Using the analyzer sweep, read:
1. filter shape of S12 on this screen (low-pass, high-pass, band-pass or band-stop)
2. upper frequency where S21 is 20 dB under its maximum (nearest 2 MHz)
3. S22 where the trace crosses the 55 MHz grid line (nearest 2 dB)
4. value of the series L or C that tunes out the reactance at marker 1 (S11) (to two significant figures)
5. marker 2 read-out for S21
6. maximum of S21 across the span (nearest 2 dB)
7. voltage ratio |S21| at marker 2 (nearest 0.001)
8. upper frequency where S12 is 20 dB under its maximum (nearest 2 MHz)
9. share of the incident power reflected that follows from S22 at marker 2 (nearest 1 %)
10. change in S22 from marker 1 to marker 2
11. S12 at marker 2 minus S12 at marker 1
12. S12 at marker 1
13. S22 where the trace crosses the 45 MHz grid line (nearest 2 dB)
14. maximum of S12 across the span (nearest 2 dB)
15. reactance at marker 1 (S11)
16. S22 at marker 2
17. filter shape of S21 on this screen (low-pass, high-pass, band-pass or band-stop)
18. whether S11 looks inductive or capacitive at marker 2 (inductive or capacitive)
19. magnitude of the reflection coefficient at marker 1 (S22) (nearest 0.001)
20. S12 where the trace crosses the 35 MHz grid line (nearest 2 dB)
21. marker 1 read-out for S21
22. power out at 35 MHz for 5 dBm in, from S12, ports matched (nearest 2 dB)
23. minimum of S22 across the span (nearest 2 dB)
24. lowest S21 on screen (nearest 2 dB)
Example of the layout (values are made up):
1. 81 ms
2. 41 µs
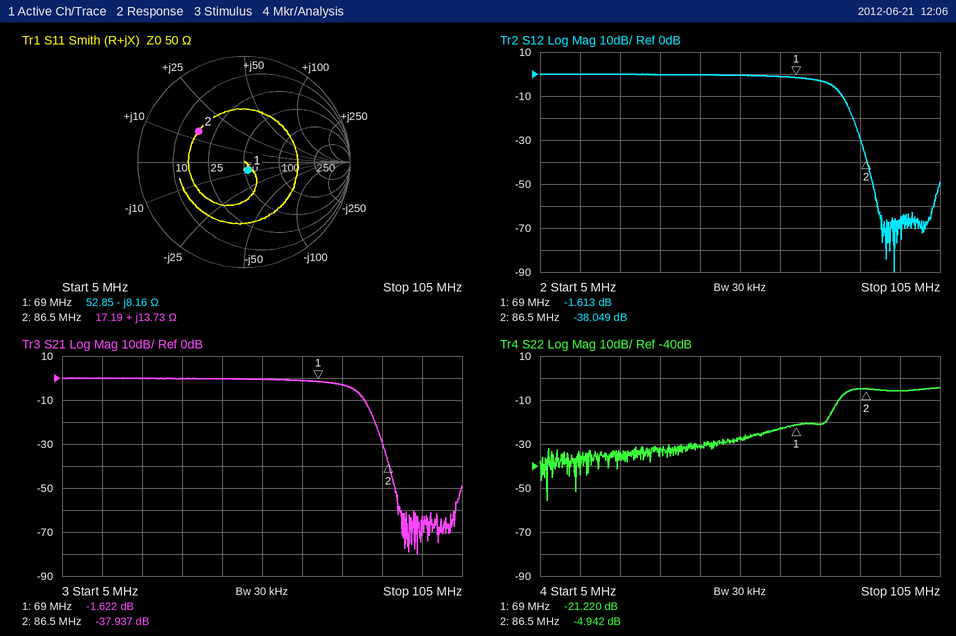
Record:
1. low-pass
2. 84 MHz
3. -28 dB
4. 19 nH
5. -37.937 dB
6. 0 dB
7. 0.013
8. 84 MHz
9. 32 %
10. 16.278 dB
11. -36.436 dB
12. -1.613 dB
13. -32 dB
14. 0 dB
15. -8.16 Ω
16. -4.942 dB
17. low-pass
18. inductive
19. 0.087
20. 0 dB
21. -1.622 dB
22. 4 dBm
23. -56 dB
24. -80 dB
